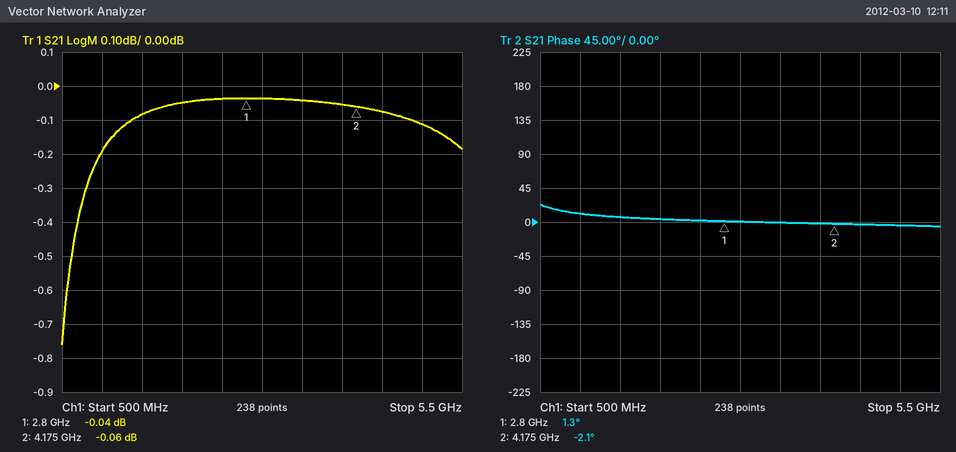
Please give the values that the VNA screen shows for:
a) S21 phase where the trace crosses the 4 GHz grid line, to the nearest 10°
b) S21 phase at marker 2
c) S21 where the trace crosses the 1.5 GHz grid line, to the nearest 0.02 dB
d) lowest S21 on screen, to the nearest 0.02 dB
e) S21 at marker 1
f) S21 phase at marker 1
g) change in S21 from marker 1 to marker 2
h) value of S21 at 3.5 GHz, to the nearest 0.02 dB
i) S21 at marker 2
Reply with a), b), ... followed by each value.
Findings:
a) 0°
b) -2.1°
c) -0.08 dB
d) -0.76 dB
e) -0.04 dB
f) 1.3°
g) -0.02 dB
h) -0.04 dB
i) -0.06 dB
